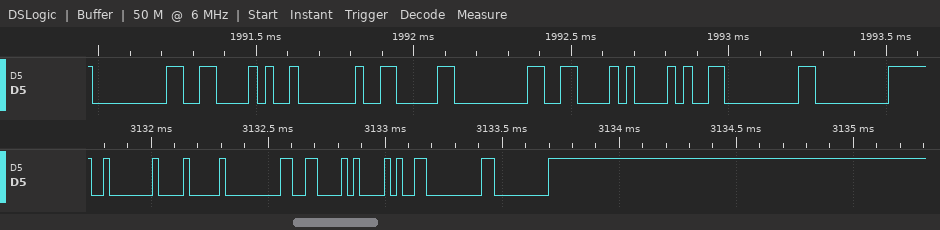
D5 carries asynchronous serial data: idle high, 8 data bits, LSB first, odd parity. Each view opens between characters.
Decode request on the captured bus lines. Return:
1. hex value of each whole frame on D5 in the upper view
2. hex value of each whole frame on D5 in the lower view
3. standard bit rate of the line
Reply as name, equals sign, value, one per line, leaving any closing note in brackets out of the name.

hex value of each whole frame on D5 in the upper view = 00, 86, 02, 06, 00, 86, 28, 00, 00
hex value of each whole frame on D5 in the lower view = 02, 08, 00, 86, 28, 00, 00
standard bit rate of the line = 38400 baud
